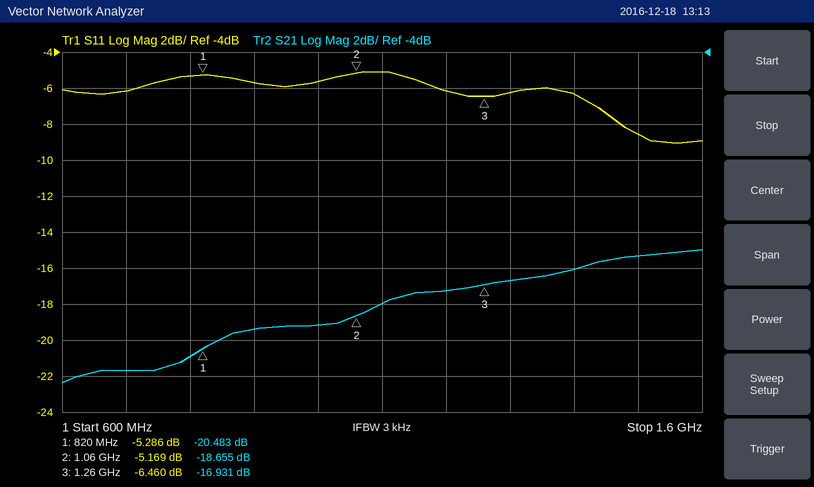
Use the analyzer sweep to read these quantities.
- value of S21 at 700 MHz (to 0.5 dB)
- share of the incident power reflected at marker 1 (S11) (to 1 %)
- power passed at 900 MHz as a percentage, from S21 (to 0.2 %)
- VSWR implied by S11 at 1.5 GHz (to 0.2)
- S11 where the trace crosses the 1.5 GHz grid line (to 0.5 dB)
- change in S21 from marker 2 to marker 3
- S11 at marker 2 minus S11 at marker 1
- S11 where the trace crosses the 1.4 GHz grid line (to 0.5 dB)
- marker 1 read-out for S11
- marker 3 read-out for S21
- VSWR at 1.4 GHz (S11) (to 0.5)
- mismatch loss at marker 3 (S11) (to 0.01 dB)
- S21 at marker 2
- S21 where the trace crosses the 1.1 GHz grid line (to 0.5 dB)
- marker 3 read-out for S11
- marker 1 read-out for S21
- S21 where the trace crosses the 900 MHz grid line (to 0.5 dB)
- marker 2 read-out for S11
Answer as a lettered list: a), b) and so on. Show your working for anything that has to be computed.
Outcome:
a) -21.5 dB
b) 10^(-5.286/10) ≈ 30 %
c) 10^(-19.5/10) ≈ 1.12 %, so 1.2 % to the nearest 0.2 %
d) |Γ| = 10^(-8.5/20) = 0.3758; VSWR = (1 + 0.3758)/(1 − 0.3758) ≈ 2.2
e) -8.5 dB
f) -16.931 − (-18.655) = 1.724 dB
g) -5.169 − (-5.286) = 0.117 dB
h) -6.5 dB
i) -5.286 dB
j) -16.931 dB
k) |Γ| = 10^(-6.5/20) = 0.4732; VSWR = (1 + 0.4732)/(1 − 0.4732) ≈ 2.80, so 3.0 to the nearest 0.5
l) −10 log10(1 − 10^(-6.46/10)) ≈ 1.11 dB
m) -18.655 dB
n) -18.0 dB
o) -6.460 dB
p) -20.483 dB
q) -19.5 dB
r) -5.169 dB
